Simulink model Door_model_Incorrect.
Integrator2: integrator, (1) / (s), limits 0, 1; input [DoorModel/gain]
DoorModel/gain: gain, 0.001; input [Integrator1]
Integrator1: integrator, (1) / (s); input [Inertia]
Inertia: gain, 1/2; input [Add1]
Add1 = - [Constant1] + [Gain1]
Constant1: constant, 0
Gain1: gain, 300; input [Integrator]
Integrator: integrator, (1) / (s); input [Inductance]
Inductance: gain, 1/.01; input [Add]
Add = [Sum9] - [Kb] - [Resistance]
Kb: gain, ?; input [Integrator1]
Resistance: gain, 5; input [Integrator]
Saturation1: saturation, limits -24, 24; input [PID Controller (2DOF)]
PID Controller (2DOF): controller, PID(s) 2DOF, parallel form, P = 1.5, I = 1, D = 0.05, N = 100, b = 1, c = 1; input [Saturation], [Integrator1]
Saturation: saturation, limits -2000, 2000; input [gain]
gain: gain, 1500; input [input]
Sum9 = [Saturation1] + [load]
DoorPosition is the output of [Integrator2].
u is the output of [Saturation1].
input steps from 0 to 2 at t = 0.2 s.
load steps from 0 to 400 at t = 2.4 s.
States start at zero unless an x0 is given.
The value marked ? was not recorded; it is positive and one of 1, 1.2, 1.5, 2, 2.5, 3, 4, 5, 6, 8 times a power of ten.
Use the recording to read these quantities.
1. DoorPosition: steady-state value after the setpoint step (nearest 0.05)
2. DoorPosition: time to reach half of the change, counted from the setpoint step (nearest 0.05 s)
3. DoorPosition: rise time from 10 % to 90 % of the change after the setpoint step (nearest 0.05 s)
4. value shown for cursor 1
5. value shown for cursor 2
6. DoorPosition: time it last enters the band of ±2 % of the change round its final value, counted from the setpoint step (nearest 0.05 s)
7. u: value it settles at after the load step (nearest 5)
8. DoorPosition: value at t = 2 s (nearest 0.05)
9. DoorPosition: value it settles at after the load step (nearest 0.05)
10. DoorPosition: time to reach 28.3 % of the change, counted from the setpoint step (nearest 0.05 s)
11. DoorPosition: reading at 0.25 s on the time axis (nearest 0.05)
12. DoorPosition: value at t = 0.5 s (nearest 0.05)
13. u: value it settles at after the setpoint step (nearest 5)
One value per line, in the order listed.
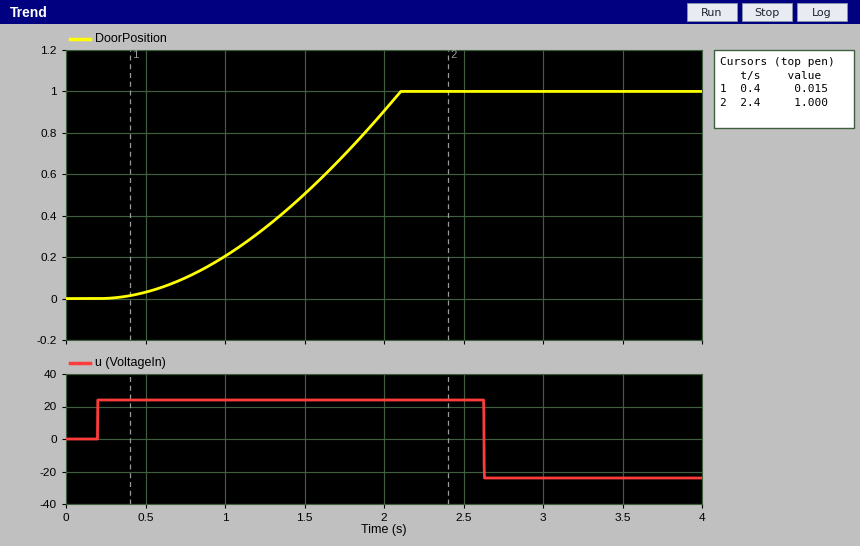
1.00
1.30 s
1.25 s
0.015
1.000
1.90 s
-25
0.90
1.00
0.95 s
0.00
0.05
25
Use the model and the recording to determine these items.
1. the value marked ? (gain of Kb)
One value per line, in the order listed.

0.015
